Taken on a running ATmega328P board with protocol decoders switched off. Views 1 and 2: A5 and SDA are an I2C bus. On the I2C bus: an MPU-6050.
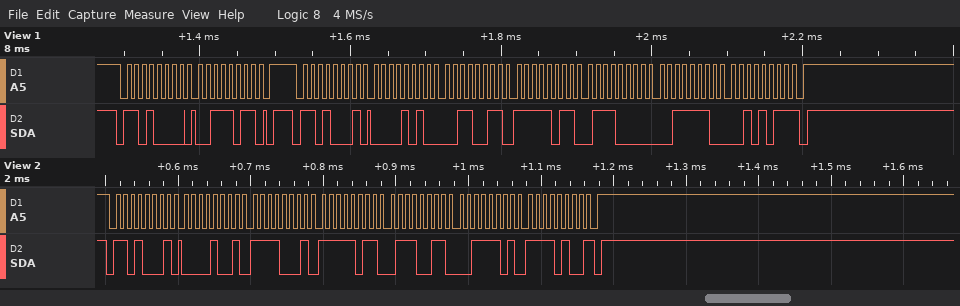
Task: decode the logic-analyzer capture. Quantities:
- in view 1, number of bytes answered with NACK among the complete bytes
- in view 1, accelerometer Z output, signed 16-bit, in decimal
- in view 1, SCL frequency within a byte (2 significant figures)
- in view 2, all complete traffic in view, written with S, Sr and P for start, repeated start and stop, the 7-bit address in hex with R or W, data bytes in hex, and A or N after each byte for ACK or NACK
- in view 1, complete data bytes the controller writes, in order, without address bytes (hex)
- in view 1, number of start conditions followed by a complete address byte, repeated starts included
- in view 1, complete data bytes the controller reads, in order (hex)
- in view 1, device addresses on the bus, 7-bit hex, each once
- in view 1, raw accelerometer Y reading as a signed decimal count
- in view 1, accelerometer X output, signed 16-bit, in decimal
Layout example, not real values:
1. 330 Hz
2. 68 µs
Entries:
1. 1
2. 15915
3. 100 kHz
4. S 68R A 09 A F1 A FB A 73 A 3D A F4 N P
5. 3B
6. 2
7. 0A 33 FB 70 3E 2B
8. 0x68
9. -1168
10. 2611
